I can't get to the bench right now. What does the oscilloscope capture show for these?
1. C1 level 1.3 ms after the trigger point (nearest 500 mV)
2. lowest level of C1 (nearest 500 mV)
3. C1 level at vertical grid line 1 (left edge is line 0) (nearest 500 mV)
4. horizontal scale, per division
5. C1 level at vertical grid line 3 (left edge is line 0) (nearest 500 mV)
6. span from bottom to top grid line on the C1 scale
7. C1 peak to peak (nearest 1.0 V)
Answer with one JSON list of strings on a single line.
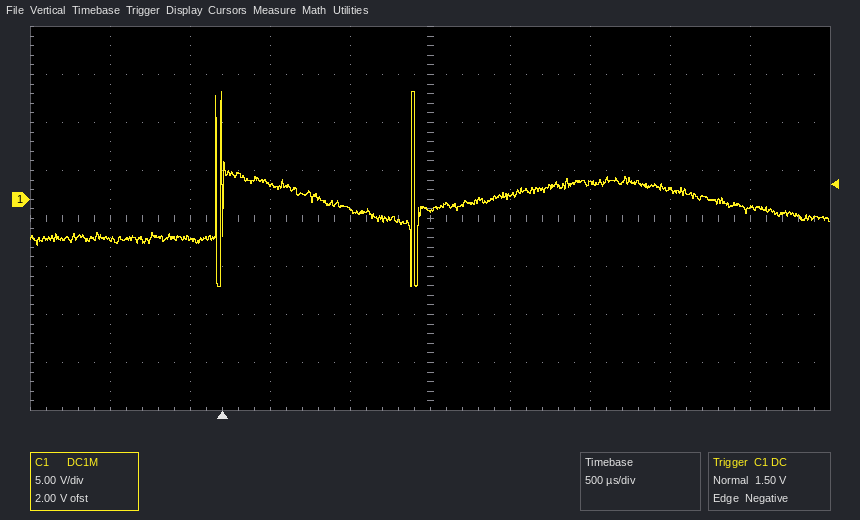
["-1.0 V", "-9.0 V", "-4.0 V", "500 µs", "1.5 V", "40 V", "20.0 V"]
